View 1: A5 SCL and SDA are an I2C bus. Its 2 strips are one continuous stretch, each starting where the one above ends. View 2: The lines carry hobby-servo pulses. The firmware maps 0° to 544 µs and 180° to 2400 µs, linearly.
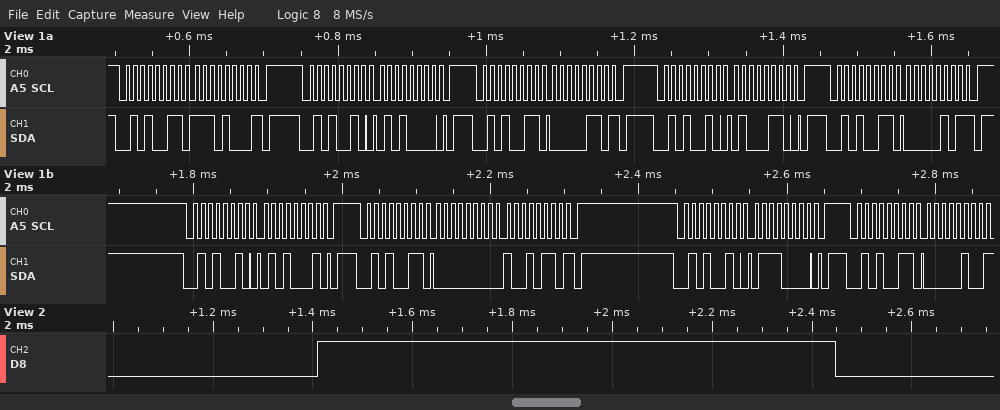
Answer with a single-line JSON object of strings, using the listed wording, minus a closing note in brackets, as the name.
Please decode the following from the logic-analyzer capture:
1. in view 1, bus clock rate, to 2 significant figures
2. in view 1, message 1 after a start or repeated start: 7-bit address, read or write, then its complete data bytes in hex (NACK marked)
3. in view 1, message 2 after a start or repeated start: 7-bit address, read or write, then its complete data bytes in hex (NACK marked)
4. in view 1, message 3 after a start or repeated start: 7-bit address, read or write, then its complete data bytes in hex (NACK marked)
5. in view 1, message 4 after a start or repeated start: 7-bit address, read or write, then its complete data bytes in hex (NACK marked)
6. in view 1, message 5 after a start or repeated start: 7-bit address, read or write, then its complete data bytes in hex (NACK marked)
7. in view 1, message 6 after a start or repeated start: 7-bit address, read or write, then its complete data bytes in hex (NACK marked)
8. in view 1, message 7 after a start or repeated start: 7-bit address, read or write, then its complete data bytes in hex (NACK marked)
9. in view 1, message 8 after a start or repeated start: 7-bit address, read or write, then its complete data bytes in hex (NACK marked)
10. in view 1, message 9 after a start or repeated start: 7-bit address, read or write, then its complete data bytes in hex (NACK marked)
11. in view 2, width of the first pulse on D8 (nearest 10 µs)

{"in view 1, bus clock rate, to 2 significant figures": "100 kHz", "in view 1, message 1 after a start or repeated start: 7-bit address, read or write, then its complete data bytes in hex": "0x29 read: E8 NACK", "in view 1, message 2 after a start or repeated start: 7-bit address, read or write, then its complete data bytes in hex": "0x29 write: 50", "in view 1, message 3 after a start or repeated start: 7-bit address, read or write, then its complete data bytes in hex": "0x29 read: 06 NACK", "in view 1, message 4 after a start or repeated start: 7-bit address, read or write, then its complete data bytes in hex": "0x29 write: 46", "in view 1, message 5 after a start or repeated start: 7-bit address, read or write, then its complete data bytes in hex": "0x29 read: 05 NACK", "in view 1, message 6 after a start or repeated start: 7-bit address, read or write, then its complete data bytes in hex": "0x29 write: 51", "in view 1, message 7 after a start or repeated start: 7-bit address, read or write, then its complete data bytes in hex": "0x29 read: 00 96 NACK", "in view 1, message 8 after a start or repeated start: 7-bit address, read or write, then its complete data bytes in hex": "0x29 write: 70", "in view 1, message 9 after a start or repeated start: 7-bit address, read or write, then its complete data bytes in hex": "0x29 read: 04 NACK", "in view 2, width of the first pulse on D8": "1040 µs"}
